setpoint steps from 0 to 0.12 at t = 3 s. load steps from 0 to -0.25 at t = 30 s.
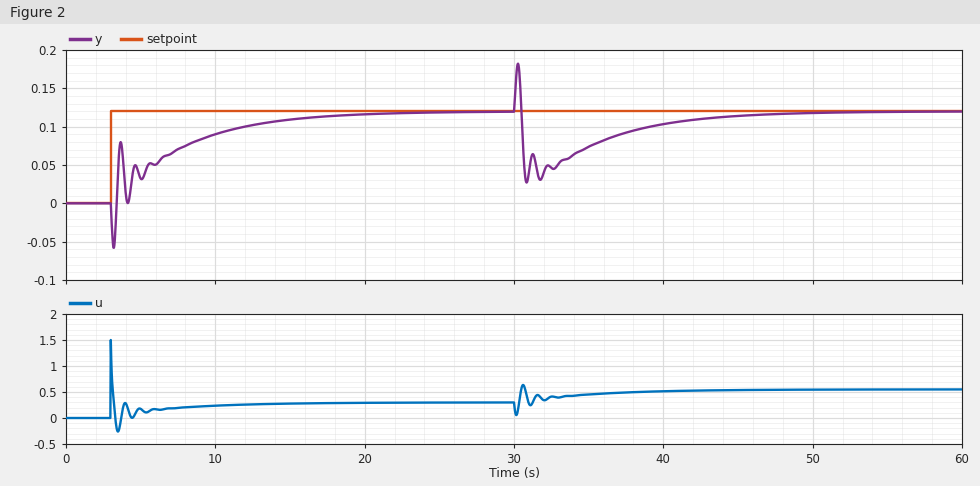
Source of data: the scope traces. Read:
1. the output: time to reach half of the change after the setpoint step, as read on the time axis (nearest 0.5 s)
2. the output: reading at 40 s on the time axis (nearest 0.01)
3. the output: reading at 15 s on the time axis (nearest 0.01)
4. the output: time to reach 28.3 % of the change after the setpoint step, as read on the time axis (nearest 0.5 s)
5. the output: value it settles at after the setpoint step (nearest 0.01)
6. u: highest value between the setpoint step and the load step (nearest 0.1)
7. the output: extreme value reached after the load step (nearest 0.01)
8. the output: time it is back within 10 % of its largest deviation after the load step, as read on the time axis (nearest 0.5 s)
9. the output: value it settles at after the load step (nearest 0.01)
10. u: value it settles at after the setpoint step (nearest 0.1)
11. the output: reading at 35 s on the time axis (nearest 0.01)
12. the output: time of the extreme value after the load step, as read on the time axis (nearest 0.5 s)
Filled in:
3.5 s
0.10
0.11
3.5 s
0.12
1.5
0.03
43.0 s
0.12
0.3
0.07
31.0 s
